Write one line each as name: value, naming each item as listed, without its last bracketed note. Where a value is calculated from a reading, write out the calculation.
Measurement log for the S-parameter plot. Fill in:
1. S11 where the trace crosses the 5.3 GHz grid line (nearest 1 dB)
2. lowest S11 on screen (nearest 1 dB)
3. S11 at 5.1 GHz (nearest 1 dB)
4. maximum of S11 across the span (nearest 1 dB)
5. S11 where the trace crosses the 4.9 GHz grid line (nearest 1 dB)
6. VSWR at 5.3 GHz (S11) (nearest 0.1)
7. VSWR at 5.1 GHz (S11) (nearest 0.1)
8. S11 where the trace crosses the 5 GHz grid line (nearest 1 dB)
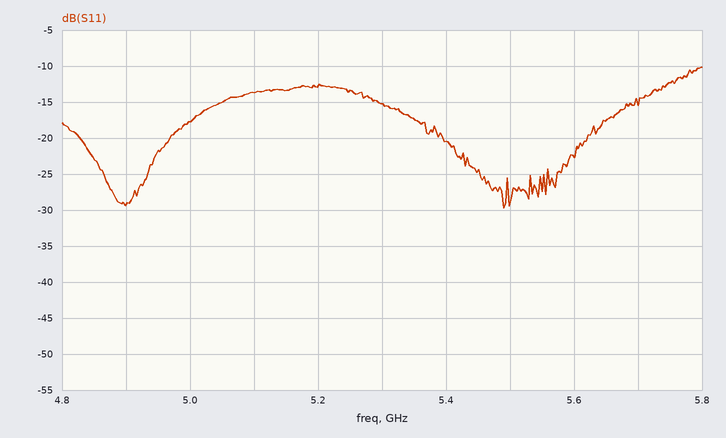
S11 where the trace crosses the 5.3 GHz grid line: -15 dB
lowest S11 on screen: -30 dB
S11 at 5.1 GHz: -14 dB
maximum of S11 across the span: -10 dB
S11 where the trace crosses the 4.9 GHz grid line: -29 dB
VSWR at 5.3 GHz (S11): |Γ| = 10^(-15/20) = 0.1778; VSWR = (1 + 0.1778)/(1 − 0.1778) ≈ 1.4
VSWR at 5.1 GHz (S11): |Γ| = 10^(-14/20) = 0.1995; VSWR = (1 + 0.1995)/(1 − 0.1995) ≈ 1.5
S11 where the trace crosses the 5 GHz grid line: -18 dB
